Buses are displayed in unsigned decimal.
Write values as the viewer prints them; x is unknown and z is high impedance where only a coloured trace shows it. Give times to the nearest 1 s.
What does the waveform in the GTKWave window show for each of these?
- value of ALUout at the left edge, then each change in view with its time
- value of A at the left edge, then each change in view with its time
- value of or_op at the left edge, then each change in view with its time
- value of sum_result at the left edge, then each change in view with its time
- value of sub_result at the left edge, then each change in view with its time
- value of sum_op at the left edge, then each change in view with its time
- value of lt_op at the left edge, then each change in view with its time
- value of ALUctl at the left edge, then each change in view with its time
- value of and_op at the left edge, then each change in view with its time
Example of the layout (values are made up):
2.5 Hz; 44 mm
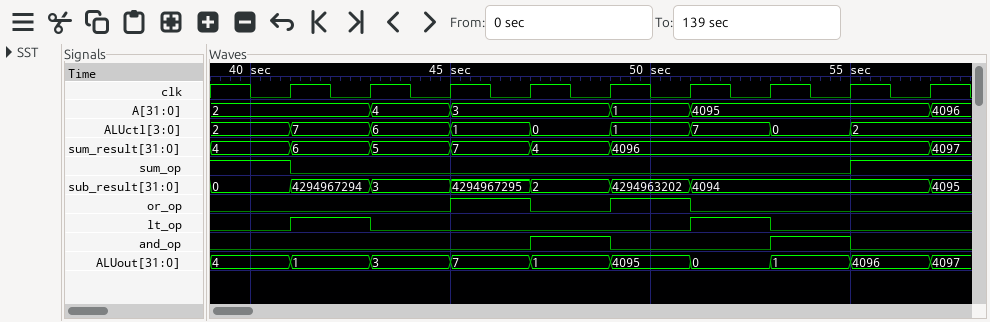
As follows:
4, 1 at 41 s, 3 at 43 s, 7 at 45 s, 1 at 47 s, 4095 at 49 s, 0 at 51 s, 1 at 53 s, 4096 at 55 s, 4097 at 57 s; 2, 4 at 43 s, 3 at 45 s, 1 at 49 s, 4095 at 51 s, 4096 at 57 s; 0, 1 at 45 s, 0 at 47 s, 1 at 49 s, 0 at 51 s; 4, 6 at 41 s, 5 at 43 s, 7 at 45 s, 4 at 47 s, 4096 at 49 s, 4097 at 57 s; 0, 4294967294 at 41 s, 3 at 43 s, 4294967295 at 45 s, 2 at 47 s, 4294963202 at 49 s, 4094 at 51 s, 4095 at 57 s; 1, 0 at 41 s, 1 at 55 s; 0, 1 at 41 s, 0 at 43 s, 1 at 51 s, 0 at 53 s; 2, 7 at 41 s, 6 at 43 s, 1 at 45 s, 0 at 47 s, 1 at 49 s, 7 at 51 s, 0 at 53 s, 2 at 55 s; 0, 1 at 47 s, 0 at 49 s, 1 at 53 s, 0 at 55 s
